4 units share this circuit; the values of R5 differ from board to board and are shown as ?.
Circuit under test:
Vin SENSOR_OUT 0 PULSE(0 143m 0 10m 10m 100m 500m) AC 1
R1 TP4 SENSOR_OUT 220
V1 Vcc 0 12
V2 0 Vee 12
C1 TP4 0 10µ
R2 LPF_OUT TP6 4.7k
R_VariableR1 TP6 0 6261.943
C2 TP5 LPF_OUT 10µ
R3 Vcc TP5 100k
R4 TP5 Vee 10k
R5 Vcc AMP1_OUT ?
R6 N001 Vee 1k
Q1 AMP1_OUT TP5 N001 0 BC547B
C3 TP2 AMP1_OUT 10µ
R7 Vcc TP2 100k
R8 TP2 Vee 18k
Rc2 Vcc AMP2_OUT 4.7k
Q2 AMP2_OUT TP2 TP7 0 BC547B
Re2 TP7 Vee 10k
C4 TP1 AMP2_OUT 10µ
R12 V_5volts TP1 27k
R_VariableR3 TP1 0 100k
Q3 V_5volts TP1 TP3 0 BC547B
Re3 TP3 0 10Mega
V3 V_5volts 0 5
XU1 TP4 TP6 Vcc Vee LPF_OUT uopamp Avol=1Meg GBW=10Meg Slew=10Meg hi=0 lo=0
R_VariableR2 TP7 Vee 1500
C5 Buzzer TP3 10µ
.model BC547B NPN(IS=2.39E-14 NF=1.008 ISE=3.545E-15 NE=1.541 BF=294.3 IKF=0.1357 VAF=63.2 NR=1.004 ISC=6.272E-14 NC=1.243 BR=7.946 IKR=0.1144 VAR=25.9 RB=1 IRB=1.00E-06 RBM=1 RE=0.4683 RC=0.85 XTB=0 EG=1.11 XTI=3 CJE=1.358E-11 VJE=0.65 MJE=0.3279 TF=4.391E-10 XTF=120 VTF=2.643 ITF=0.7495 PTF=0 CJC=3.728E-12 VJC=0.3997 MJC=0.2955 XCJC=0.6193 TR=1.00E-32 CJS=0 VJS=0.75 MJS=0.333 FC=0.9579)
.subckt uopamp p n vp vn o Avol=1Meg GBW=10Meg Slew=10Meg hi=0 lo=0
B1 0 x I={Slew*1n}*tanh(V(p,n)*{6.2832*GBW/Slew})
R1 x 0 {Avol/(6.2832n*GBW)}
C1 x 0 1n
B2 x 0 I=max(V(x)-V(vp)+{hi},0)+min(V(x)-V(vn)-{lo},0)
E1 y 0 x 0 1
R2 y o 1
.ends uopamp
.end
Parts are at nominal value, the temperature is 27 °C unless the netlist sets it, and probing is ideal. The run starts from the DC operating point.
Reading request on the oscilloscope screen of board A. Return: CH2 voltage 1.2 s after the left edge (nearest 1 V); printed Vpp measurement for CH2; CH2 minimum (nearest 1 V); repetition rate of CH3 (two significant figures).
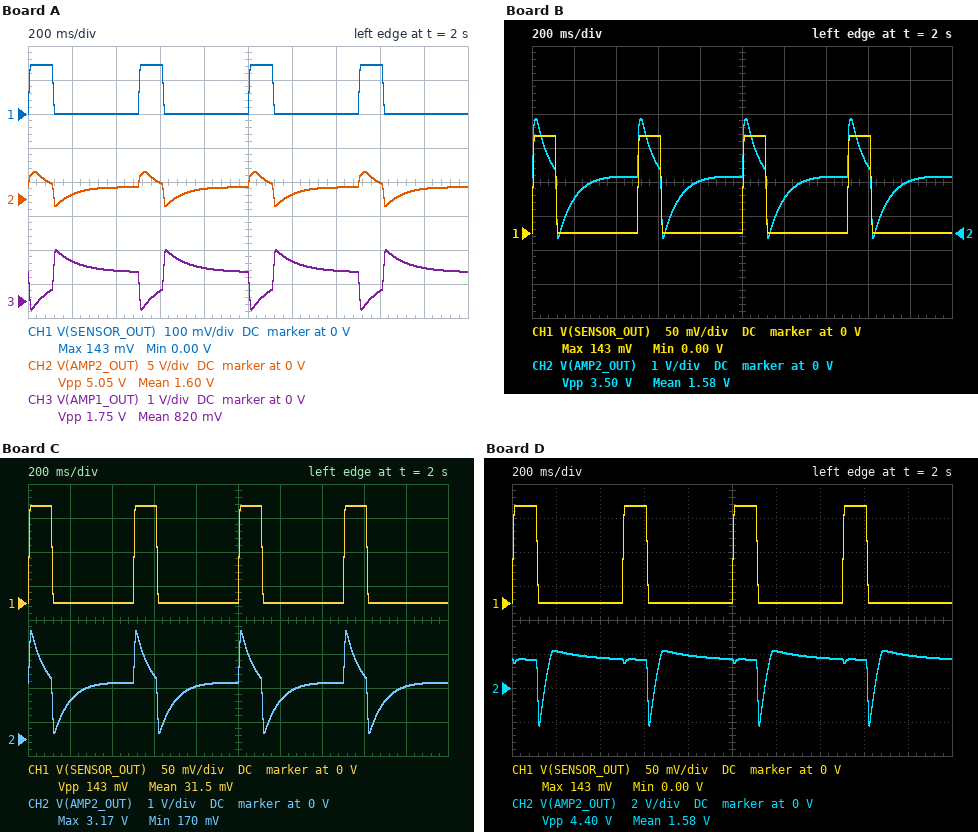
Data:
1 V
5.05 V
-1 V
2.0 Hz
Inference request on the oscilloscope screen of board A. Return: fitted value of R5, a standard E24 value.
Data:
7.5 kΩ
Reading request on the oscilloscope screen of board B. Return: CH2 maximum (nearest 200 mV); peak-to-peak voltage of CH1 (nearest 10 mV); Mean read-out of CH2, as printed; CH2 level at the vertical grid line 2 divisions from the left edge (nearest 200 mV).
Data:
3.4 V
140 mV
1.58 V
1.6 V
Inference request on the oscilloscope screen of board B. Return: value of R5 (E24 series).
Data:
3.9 kΩ
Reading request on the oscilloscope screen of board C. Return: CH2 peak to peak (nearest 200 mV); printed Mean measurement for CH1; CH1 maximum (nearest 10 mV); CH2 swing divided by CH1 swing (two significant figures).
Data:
3.0 V
31.5 mV
140 mV
21
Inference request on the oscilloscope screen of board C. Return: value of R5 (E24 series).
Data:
3 kΩ
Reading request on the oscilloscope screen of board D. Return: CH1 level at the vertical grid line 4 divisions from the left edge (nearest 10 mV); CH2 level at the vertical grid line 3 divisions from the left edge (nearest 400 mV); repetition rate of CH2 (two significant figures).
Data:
0 V
1.6 V
2.0 Hz
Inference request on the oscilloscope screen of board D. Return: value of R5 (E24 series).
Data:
18 kΩ
